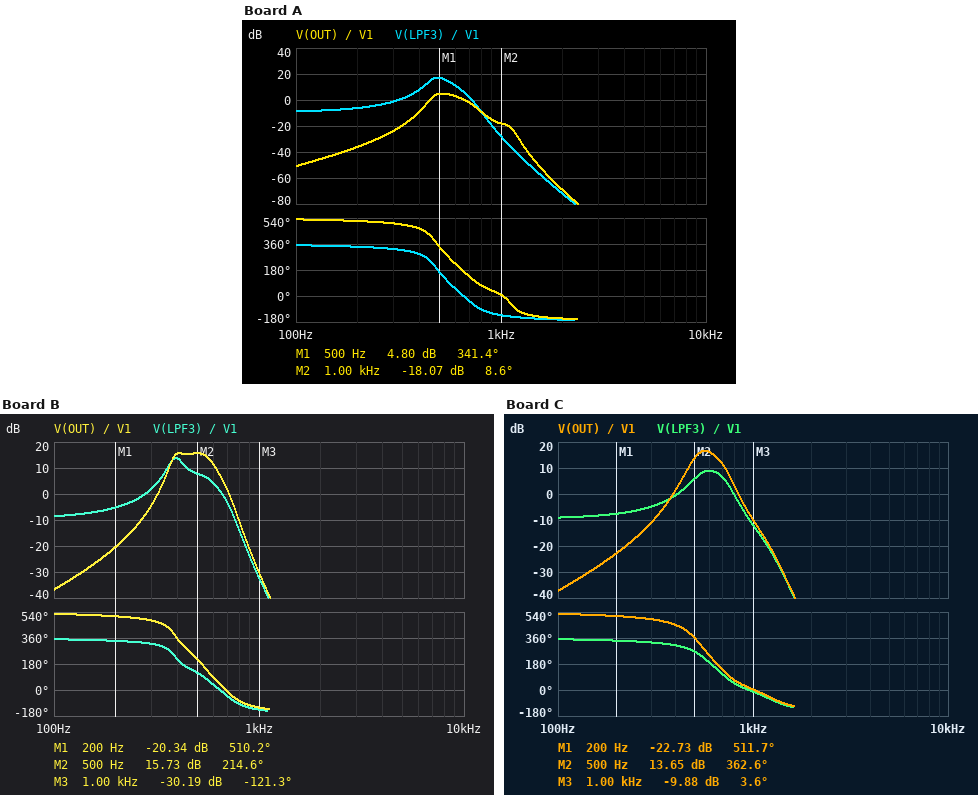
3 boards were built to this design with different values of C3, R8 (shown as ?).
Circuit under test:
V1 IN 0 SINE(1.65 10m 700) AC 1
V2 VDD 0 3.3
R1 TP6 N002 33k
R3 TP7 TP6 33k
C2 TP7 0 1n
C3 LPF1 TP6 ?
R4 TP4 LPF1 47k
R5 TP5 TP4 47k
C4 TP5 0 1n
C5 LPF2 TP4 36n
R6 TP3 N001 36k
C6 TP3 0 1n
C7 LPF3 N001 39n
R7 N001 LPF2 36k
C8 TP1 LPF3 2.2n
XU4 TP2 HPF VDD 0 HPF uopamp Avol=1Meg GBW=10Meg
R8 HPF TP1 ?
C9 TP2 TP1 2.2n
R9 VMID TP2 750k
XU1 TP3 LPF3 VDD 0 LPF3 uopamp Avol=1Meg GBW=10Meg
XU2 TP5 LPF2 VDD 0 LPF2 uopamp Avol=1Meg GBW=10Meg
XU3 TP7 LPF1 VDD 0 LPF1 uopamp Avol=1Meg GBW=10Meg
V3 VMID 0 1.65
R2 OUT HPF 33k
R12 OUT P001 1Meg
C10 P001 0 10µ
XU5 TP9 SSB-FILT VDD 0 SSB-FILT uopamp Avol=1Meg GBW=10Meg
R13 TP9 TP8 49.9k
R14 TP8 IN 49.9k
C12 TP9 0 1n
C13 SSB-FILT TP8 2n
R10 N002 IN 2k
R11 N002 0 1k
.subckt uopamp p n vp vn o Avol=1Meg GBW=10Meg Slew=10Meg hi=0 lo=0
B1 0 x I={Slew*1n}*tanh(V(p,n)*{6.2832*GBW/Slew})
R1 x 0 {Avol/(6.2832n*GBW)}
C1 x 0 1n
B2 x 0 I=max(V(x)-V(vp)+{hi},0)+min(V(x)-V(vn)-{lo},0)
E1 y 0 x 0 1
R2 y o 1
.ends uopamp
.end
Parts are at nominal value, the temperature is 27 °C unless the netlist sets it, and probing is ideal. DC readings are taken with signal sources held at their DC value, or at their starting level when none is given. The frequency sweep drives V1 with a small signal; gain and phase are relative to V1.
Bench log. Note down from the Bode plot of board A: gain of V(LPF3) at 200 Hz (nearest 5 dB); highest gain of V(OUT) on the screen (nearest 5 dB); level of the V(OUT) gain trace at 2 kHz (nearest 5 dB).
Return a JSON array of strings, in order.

["-5 dB", "5 dB", "-70 dB"]
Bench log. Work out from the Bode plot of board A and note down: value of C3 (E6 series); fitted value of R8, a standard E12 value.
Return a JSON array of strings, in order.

["100 nF", "5.6 kΩ"]
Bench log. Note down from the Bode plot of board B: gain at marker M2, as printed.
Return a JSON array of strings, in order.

["15.73 dB"]
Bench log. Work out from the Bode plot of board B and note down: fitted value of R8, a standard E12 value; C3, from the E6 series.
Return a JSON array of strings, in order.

["27 kΩ", "150 nF"]
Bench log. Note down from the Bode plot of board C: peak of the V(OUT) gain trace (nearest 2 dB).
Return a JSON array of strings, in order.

["16 dB"]
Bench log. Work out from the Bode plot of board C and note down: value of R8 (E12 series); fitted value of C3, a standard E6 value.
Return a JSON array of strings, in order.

["27 kΩ", "15 nF"]
